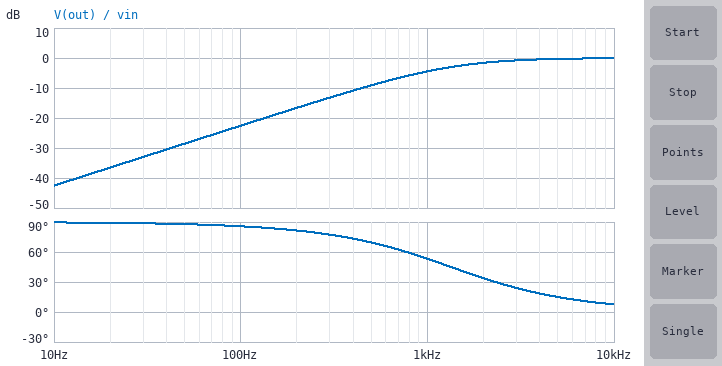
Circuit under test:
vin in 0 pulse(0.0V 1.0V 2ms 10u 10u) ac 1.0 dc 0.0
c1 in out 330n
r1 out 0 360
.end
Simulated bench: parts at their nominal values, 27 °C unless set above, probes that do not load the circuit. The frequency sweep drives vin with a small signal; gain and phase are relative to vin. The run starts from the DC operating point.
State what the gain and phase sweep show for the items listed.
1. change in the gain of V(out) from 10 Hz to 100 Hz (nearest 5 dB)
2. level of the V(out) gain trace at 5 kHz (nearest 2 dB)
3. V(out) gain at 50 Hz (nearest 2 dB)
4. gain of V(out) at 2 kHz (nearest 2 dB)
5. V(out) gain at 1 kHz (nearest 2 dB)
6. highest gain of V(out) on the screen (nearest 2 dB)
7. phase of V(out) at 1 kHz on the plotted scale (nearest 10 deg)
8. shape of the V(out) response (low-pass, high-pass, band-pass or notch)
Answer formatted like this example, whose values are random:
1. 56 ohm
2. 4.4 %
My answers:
1. 20 dB
2. 0 dB
3. -28 dB
4. -2 dB
5. -4 dB
6. 0 dB
7. 50 deg
8. high-pass
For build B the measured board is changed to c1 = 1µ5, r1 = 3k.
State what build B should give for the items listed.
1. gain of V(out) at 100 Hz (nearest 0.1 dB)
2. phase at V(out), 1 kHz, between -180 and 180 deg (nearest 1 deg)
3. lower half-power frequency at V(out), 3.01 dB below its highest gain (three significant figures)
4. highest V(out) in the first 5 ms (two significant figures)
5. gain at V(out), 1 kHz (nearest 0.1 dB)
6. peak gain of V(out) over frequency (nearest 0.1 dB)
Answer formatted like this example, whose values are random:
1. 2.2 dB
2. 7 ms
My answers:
1. -0.5 dB
2. 2 deg
3. 35.4 Hz
4. 1.0 V
5. 0 dB
6. 0 dB
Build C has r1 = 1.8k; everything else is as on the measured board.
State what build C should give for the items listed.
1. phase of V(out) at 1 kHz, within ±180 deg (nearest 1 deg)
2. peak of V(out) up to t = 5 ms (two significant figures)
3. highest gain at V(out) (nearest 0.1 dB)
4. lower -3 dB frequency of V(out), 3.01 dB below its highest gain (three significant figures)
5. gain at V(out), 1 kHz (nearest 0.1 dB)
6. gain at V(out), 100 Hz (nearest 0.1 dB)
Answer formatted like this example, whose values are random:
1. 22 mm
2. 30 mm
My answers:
1. 15 deg
2. 990 mV
3. 0 dB
4. 268 Hz
5. -0.3 dB
6. -9.1 dB
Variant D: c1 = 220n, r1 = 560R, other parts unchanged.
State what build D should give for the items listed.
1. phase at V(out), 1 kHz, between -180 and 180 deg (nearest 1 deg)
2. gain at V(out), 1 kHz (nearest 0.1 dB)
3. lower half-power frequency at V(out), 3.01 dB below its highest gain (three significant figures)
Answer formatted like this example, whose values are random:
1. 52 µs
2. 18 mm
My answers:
1. 52 deg
2. -4.3 dB
3. 1.29 kHz
